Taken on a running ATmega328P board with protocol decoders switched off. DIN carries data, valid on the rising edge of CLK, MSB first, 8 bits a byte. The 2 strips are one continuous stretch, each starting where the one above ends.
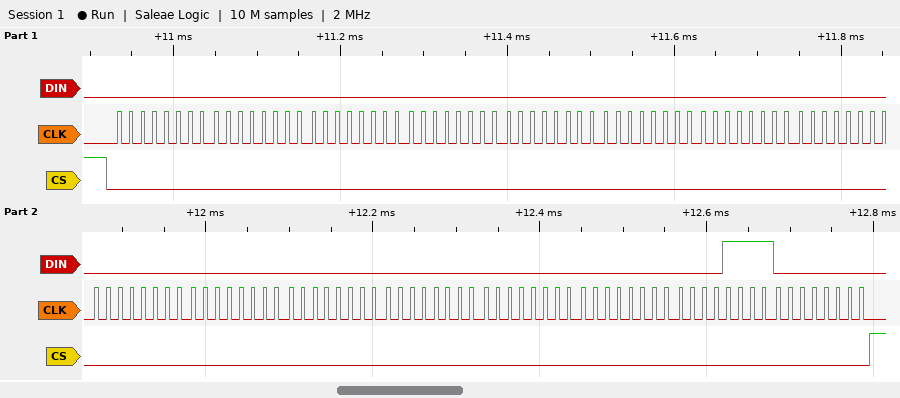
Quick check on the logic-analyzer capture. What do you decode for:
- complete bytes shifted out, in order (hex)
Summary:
00 00 00 00 00 00 00 00 00 00 00 00 00 00 0F 00
